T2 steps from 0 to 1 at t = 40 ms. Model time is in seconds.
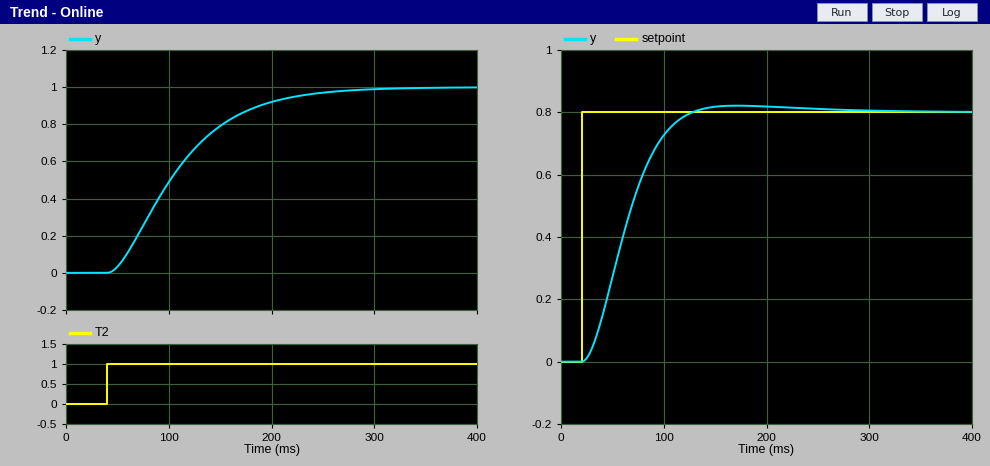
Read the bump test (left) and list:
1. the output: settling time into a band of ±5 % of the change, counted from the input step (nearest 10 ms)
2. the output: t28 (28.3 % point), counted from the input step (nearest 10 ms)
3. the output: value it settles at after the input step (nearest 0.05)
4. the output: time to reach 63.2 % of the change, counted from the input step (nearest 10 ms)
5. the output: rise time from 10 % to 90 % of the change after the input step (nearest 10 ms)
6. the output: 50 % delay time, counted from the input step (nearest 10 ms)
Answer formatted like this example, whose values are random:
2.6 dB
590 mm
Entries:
180 ms
40 ms
1.00
80 ms
130 ms
60 ms
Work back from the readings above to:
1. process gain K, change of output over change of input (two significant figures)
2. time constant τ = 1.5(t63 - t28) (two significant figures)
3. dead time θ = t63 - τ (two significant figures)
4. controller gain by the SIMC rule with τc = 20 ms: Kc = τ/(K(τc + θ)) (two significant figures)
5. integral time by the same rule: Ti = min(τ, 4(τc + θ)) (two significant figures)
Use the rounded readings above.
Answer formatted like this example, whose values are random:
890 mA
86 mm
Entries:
1.0
60 ms
20 ms
1.5
60 ms
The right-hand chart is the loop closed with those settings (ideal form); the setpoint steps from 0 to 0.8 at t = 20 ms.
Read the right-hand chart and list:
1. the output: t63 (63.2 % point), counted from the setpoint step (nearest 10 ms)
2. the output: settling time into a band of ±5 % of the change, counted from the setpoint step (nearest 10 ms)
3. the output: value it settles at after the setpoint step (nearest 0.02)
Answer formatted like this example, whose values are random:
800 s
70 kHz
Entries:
50 ms
90 ms
0.80
